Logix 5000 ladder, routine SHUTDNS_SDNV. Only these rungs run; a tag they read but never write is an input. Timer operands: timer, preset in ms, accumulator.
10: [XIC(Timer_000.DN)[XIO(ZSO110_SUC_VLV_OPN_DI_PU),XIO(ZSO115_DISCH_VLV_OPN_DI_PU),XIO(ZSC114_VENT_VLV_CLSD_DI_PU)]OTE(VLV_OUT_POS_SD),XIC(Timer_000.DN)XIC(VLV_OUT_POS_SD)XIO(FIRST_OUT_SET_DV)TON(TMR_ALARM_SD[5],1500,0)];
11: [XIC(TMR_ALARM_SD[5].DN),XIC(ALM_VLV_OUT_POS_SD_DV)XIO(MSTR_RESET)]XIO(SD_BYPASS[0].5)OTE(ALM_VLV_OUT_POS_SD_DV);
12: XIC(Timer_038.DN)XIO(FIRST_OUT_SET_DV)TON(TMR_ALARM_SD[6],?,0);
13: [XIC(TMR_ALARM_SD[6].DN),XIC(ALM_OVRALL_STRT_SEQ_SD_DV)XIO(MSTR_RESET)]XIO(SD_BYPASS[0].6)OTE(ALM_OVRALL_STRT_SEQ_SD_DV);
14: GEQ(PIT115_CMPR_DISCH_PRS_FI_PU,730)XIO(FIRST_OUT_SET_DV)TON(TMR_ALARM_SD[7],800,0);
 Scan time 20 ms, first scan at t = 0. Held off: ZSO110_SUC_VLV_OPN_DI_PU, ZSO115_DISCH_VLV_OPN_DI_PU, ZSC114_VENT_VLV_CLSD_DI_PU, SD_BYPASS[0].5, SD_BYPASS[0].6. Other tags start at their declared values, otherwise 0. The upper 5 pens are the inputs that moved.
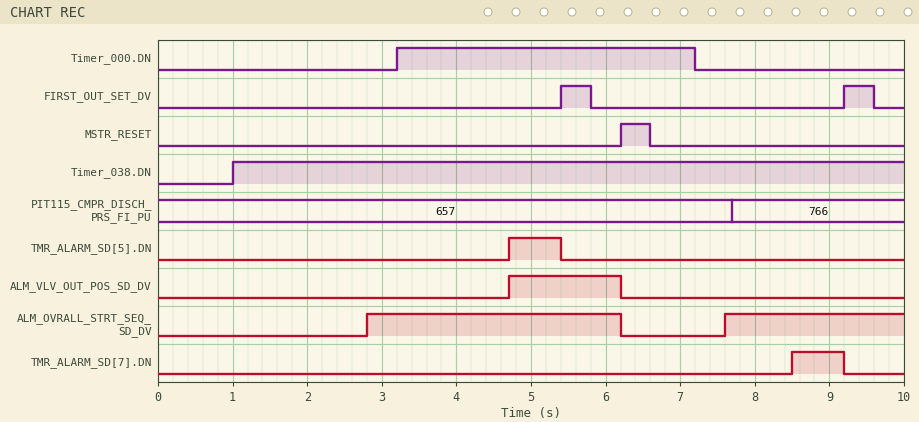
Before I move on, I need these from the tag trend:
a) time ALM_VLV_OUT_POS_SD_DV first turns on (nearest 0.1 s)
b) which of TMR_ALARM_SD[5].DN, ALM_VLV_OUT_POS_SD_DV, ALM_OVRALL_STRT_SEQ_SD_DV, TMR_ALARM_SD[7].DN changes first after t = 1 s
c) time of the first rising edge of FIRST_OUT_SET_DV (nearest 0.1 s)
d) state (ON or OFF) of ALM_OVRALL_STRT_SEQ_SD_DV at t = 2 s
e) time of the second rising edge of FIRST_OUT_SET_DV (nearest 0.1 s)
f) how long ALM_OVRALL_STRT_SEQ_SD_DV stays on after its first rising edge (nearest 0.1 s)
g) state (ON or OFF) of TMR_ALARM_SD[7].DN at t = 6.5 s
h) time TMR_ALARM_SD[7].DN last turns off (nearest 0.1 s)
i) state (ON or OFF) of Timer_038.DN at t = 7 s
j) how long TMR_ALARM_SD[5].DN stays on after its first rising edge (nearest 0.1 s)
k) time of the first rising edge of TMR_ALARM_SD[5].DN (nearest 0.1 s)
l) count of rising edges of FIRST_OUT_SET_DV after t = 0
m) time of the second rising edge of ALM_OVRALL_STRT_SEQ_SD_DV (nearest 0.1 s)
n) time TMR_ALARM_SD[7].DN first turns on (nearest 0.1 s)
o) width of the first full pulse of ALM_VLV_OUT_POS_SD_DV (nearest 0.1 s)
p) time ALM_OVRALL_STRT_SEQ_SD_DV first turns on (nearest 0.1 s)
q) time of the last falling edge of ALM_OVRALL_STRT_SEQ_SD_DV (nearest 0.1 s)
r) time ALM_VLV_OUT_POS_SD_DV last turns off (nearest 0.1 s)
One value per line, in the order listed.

4.7 s
ALM_OVRALL_STRT_SEQ_SD_DV
5.4 s
OFF
9.2 s
3.4 s
OFF
9.2 s
ON
0.7 s
4.7 s
2
7.6 s
8.5 s
1.5 s
2.8 s
6.2 s
6.2 s
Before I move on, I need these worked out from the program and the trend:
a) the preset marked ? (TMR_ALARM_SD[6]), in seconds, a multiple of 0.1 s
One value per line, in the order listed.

1.8 s
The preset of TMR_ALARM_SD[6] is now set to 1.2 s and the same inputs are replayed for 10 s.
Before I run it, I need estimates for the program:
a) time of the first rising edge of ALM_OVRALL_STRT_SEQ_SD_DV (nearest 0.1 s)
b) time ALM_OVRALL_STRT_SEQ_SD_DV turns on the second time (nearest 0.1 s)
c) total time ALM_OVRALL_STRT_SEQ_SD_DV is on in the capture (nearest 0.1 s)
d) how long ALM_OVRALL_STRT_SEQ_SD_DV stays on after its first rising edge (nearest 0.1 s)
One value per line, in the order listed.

2.2 s
7.0 s
7.0 s
4.0 s
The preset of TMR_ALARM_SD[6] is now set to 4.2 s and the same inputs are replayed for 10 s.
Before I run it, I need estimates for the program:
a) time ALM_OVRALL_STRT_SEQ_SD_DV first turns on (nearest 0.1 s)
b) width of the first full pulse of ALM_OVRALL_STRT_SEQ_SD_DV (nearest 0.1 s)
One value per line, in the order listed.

5.2 s
1.0 s
